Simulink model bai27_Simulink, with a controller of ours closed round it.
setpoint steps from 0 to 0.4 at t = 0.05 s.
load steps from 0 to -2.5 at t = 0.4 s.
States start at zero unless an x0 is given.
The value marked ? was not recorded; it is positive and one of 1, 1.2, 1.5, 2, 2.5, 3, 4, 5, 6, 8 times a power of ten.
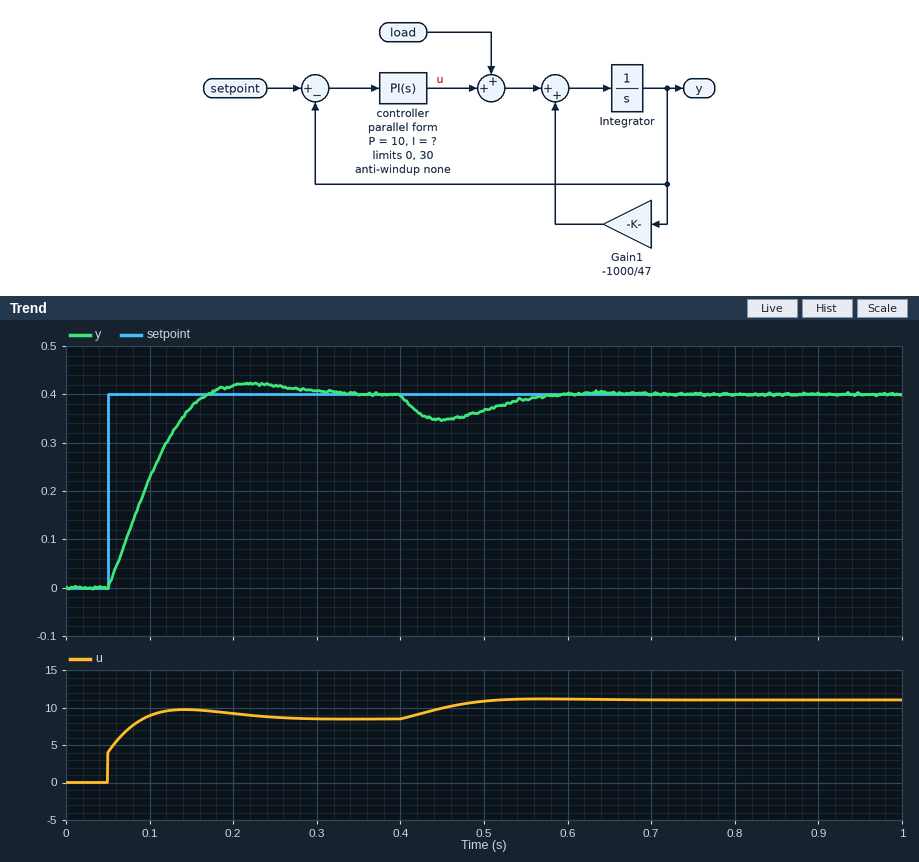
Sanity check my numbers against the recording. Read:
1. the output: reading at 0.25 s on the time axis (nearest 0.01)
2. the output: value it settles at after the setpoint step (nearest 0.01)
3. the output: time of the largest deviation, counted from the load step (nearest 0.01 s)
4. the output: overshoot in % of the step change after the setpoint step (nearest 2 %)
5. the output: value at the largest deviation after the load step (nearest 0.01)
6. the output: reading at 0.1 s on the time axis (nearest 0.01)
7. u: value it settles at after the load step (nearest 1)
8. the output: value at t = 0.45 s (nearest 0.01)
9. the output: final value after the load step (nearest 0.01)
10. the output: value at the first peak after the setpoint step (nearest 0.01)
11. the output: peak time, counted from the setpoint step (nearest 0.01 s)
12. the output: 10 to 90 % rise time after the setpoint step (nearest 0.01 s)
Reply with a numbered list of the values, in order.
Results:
1. 0.42
2. 0.40
3. 0.05 s
4. 6 %
5. 0.35
6. 0.23
7. 11
8. 0.35
9. 0.40
10. 0.42
11. 0.17 s
12. 0.08 s
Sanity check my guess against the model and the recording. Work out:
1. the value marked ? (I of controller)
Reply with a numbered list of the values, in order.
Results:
1. 500
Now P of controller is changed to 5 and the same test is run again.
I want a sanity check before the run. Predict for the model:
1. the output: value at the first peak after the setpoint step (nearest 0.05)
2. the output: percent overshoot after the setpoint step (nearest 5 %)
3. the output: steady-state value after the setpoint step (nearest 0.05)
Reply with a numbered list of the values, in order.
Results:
1. 0.45
2. 10 %
3. 0.40
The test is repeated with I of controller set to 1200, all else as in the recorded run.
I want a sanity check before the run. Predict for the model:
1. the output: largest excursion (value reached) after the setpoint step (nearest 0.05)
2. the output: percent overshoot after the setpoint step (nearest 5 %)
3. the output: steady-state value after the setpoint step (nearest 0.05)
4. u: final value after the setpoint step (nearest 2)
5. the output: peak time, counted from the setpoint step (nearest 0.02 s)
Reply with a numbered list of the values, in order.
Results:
1. 0.50
2. 20 %
3. 0.40
4. 8
5. 0.10 s
